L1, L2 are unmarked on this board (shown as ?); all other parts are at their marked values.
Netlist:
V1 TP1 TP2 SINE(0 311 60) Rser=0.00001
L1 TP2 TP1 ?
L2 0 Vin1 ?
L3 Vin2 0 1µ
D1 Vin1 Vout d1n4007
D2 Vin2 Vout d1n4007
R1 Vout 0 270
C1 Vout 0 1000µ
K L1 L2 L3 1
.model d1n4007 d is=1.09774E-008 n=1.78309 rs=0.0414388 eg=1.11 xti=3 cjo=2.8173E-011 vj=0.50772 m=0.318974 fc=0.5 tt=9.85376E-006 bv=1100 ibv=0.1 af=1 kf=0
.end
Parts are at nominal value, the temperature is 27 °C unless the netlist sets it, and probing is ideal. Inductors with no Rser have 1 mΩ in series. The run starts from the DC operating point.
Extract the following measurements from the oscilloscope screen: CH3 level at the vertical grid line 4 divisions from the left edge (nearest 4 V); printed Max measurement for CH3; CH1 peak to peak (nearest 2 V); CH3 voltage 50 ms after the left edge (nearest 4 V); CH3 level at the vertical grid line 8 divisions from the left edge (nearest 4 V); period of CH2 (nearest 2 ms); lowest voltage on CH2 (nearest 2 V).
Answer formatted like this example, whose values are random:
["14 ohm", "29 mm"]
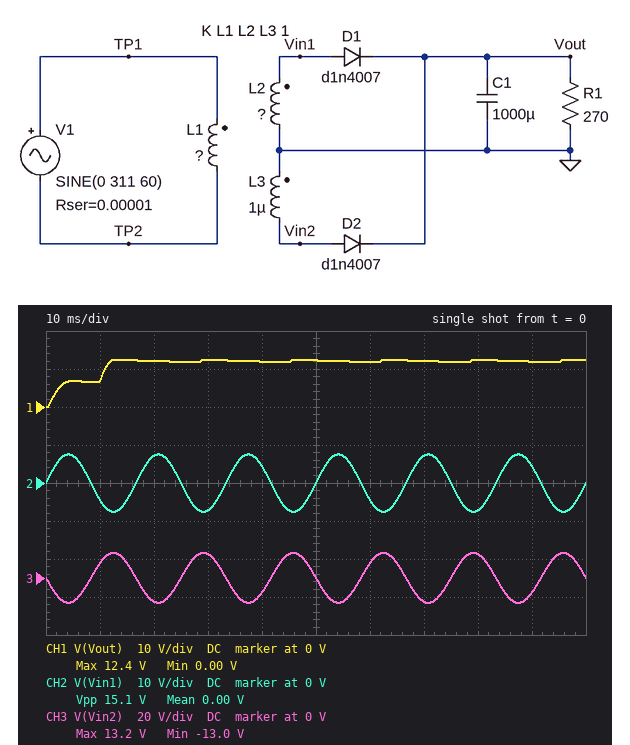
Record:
["-8 V", "13.2 V", "12 V", "0 V", "12 V", "16 ms", "-8 V"]
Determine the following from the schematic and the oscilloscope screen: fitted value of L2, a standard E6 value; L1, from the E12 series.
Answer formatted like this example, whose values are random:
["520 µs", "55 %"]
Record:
["330 nH", "560 µH"]
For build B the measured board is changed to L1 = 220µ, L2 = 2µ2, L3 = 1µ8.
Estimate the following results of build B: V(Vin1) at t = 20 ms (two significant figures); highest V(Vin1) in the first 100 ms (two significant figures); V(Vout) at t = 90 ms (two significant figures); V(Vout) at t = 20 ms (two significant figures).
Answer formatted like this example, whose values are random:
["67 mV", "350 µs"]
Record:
["29 V", "31 V", "30 V", "28 V"]
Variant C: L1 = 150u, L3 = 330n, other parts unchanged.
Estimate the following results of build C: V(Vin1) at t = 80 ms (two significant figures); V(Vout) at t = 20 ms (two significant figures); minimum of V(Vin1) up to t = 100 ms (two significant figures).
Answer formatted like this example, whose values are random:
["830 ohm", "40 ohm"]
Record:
["-14 V", "14 V", "-15 V"]
